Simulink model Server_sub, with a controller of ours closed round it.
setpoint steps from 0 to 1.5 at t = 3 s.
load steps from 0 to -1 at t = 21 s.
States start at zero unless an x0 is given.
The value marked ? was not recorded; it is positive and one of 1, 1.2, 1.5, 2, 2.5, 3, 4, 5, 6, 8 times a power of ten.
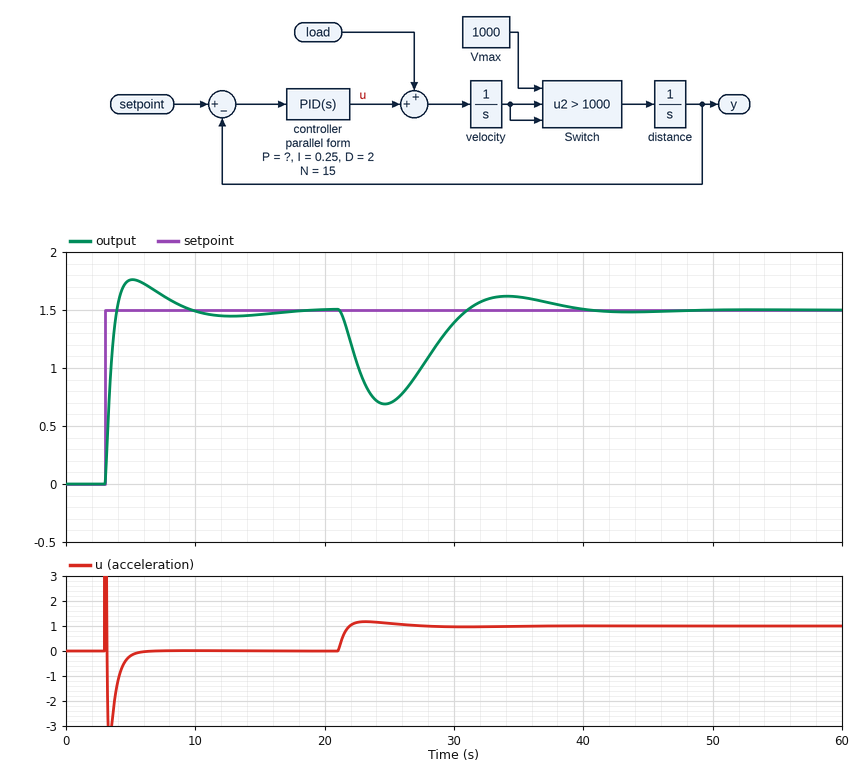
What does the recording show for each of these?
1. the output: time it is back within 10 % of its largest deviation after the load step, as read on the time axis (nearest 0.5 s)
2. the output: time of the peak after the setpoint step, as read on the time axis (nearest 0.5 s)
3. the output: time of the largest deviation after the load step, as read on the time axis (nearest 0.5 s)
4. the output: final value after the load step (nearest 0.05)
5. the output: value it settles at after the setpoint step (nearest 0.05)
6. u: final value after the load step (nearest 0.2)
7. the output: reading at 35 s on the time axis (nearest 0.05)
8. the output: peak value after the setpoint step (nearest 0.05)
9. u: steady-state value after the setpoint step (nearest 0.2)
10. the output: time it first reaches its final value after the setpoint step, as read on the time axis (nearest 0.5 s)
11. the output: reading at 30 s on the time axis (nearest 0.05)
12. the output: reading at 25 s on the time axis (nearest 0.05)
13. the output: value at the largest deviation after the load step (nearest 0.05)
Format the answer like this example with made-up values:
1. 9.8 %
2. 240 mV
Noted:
1. 36.5 s
2. 5.0 s
3. 24.5 s
4. 1.50
5. 1.50
6. 1.0
7. 1.60
8. 1.75
9. 0.0
10. 4.0 s
11. 1.40
12. 0.70
13. 0.70
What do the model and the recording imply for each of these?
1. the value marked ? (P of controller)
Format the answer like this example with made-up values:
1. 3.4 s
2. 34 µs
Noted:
1. 0.8
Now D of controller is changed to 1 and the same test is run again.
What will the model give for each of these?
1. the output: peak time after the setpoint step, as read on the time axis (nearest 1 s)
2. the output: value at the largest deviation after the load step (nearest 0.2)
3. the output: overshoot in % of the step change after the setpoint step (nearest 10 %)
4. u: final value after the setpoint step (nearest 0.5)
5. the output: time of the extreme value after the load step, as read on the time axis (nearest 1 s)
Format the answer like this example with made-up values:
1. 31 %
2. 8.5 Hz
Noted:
1. 6 s
2. 0.4
3. 40 %
4. 0.0
5. 24 s
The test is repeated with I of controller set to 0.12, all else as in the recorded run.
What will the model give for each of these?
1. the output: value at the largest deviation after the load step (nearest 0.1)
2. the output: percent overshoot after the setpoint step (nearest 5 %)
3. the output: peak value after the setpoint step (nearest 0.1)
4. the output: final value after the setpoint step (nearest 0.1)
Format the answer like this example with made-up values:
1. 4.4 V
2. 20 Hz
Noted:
1. 0.6
2. 15 %
3. 1.7
4. 1.5
